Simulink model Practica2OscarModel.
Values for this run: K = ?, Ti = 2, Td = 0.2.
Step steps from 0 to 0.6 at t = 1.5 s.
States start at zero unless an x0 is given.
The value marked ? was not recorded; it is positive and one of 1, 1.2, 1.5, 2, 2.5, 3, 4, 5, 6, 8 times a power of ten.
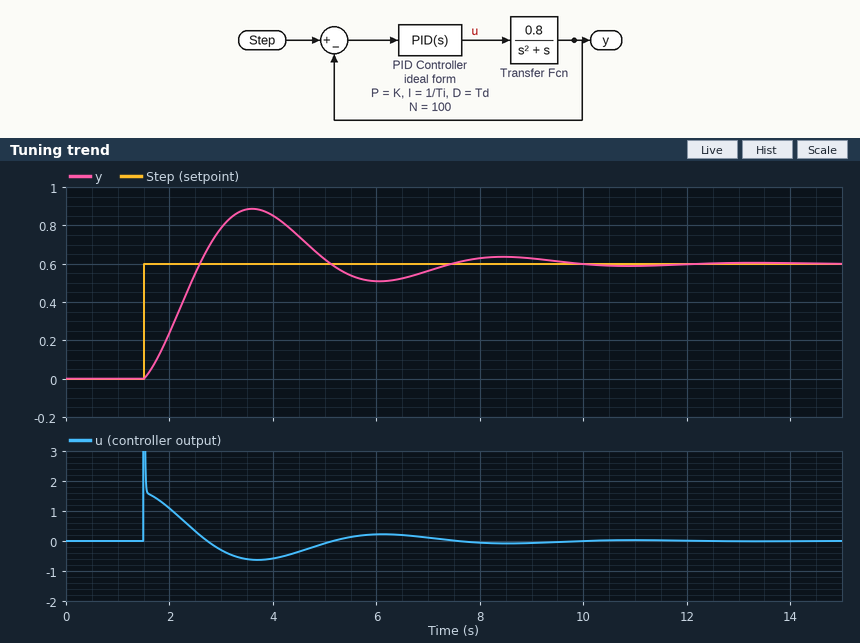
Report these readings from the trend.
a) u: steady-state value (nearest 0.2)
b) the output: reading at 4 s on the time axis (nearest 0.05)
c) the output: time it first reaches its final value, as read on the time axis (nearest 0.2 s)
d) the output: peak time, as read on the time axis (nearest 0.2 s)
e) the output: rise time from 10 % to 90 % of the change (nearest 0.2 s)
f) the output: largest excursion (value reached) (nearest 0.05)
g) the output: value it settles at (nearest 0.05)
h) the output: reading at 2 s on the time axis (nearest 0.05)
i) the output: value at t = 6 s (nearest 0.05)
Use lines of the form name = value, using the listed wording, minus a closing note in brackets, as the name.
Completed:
u: steady-state value = 0.0
the output: reading at 4 s on the time axis = 0.85
the output: time it first reaches its final value, as read on the time axis = 2.6 s
the output: peak time, as read on the time axis = 3.6 s
the output: rise time from 10 % to 90 % of the change = 0.8 s
the output: largest excursion (value reached) = 0.90
the output: value it settles at = 0.60
the output: reading at 2 s on the time axis = 0.25
the output: value at t = 6 s = 0.50
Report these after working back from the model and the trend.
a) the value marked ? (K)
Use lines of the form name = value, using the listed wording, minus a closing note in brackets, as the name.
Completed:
the value marked ? = 3
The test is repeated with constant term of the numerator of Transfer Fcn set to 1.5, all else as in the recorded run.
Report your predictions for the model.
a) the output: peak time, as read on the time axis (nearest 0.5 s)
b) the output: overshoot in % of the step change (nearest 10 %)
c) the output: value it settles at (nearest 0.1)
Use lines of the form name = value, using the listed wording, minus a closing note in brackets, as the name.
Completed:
the output: peak time, as read on the time axis = 3.0 s
the output: overshoot in % of the step change = 40 %
the output: value it settles at = 0.6
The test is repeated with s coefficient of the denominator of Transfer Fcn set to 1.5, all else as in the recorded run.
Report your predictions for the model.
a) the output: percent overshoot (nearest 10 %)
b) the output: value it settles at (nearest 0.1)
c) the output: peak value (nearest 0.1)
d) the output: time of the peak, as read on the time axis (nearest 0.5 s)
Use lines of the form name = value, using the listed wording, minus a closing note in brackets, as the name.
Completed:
the output: percent overshoot = 40 %
the output: value it settles at = 0.6
the output: peak value = 0.8
the output: time of the peak, as read on the time axis = 4.0 s
